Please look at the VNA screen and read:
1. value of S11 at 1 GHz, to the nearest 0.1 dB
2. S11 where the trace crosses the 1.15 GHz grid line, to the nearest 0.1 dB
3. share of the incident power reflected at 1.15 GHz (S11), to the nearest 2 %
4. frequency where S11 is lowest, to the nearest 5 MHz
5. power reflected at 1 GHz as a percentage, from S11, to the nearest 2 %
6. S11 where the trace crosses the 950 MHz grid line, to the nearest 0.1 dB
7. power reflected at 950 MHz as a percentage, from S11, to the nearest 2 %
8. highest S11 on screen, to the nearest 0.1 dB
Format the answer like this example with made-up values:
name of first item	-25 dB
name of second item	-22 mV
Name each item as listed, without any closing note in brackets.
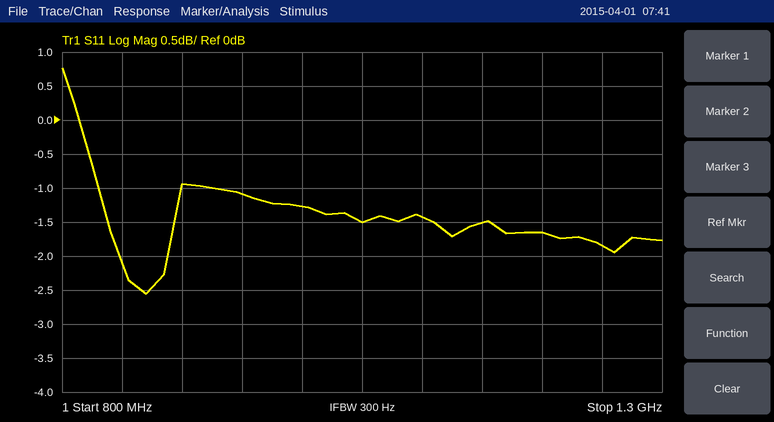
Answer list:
value of S11 at 1 GHz, to the nearest 0.1 dB	-1.3 dB
S11 where the trace crosses the 1.15 GHz grid line, to the nearest 0.1 dB	-1.5 dB
share of the incident power reflected at 1.15 GHz (S11), to the nearest 2 %	70 %
frequency where S11 is lowest, to the nearest 5 MHz	870 MHz
power reflected at 1 GHz as a percentage, from S11, to the nearest 2 %	74 %
S11 where the trace crosses the 950 MHz grid line, to the nearest 0.1 dB	-1.1 dB
power reflected at 950 MHz as a percentage, from S11, to the nearest 2 %	78 %
highest S11 on screen, to the nearest 0.1 dB	0.8 dB
